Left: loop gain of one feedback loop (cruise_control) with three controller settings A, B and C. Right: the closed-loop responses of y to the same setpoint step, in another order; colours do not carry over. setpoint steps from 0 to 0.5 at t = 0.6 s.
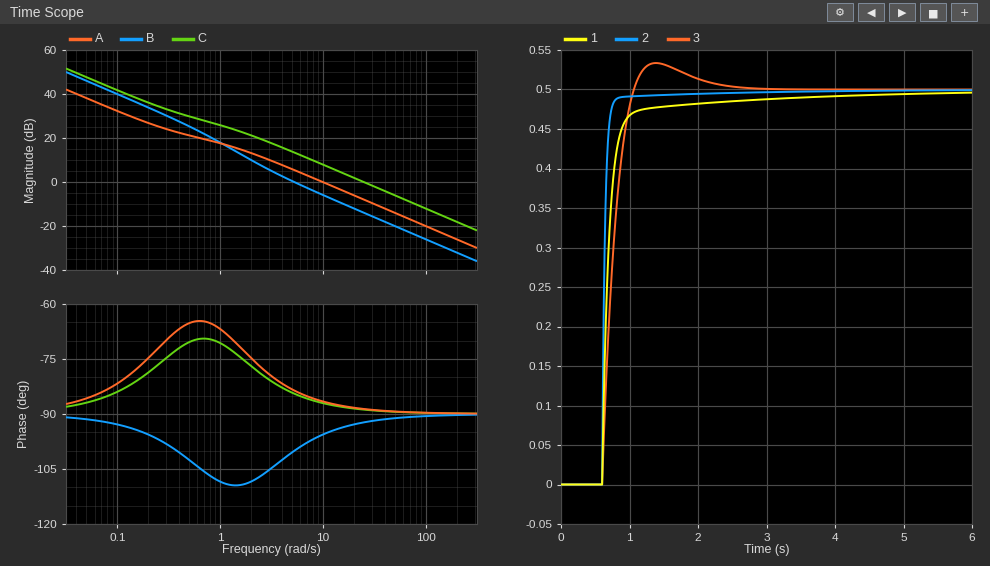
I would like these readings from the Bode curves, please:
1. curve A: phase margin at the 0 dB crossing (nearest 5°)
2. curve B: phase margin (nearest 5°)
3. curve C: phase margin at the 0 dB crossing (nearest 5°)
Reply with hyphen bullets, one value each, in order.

- 95°
- 80°
- 90°
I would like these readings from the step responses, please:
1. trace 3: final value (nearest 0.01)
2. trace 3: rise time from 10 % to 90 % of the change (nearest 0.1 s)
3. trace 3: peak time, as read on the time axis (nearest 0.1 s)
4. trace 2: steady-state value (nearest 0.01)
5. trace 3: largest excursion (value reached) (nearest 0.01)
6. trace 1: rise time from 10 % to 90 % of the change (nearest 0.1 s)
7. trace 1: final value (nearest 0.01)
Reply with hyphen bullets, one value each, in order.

- 0.50
- 0.3 s
- 1.4 s
- 0.50
- 0.53
- 0.3 s
- 0.50
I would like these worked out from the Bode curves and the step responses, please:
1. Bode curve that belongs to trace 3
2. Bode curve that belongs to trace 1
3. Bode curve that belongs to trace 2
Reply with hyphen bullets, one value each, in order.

- B
- A
- C
